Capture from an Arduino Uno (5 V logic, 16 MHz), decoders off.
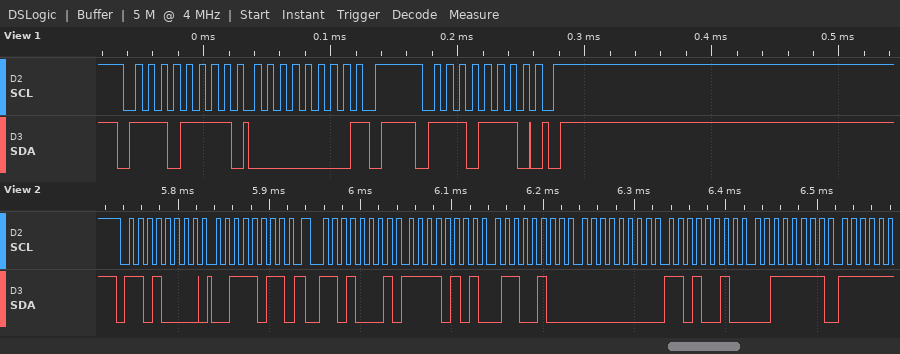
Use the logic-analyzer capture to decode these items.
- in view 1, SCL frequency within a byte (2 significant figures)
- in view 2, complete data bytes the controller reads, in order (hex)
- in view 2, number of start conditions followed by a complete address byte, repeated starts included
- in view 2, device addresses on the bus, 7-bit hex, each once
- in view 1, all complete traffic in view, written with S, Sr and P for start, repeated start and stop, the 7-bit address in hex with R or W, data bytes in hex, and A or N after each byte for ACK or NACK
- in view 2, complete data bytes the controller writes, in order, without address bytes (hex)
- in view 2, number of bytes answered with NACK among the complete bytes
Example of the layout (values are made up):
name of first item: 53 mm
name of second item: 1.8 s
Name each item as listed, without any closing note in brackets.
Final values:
in view 1, SCL frequency within a byte: 100 kHz
in view 2, complete data bytes the controller reads, in order: F5 64 00 D2 3F
in view 2, number of start conditions followed by a complete address byte, repeated starts included: 2
in view 2, device addresses on the bus, 7-bit hex, each once: 0x68
in view 1, all complete traffic in view, written with S, Sr and P for start, repeated start and stop, the 7-bit address in hex with R or W, data bytes in hex, and A or N after each byte for ACK or NACK: S 77R A 00 N P S 77W A P
in view 2, complete data bytes the controller writes, in order, without address bytes: 3B
in view 2, number of bytes answered with NACK among the complete bytes: 0
